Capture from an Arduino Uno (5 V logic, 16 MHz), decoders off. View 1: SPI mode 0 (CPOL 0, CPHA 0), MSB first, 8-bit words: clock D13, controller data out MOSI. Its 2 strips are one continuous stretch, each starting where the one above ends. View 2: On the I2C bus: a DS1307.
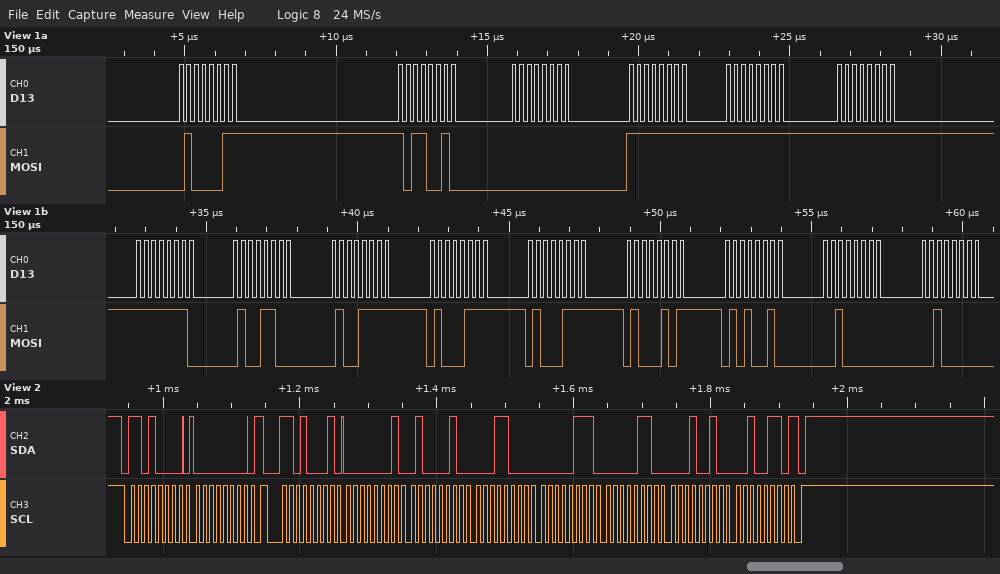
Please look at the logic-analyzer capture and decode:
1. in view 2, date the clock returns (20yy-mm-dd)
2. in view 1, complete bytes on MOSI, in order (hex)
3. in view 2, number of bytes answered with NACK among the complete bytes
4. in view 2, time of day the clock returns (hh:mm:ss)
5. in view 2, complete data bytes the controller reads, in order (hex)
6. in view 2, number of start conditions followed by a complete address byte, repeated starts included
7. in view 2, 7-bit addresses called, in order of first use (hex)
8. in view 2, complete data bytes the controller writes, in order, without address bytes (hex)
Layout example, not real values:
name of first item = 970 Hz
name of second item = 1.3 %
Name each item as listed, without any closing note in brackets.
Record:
in view 2, date the clock returns = 2026-12-06
in view 1, complete bytes on MOSI, in order = 43 B2 00 FF FF FF FE 4C 4F 47 47 45 52 20 20
in view 2, number of bytes answered with NACK among the complete bytes = 1
in view 2, time of day the clock returns = 18:42:01
in view 2, complete data bytes the controller reads, in order = 01 42 18 07 06 12 26
in view 2, number of start conditions followed by a complete address byte, repeated starts included = 2
in view 2, 7-bit addresses called, in order of first use = 0x68
in view 2, complete data bytes the controller writes, in order, without address bytes = 00
